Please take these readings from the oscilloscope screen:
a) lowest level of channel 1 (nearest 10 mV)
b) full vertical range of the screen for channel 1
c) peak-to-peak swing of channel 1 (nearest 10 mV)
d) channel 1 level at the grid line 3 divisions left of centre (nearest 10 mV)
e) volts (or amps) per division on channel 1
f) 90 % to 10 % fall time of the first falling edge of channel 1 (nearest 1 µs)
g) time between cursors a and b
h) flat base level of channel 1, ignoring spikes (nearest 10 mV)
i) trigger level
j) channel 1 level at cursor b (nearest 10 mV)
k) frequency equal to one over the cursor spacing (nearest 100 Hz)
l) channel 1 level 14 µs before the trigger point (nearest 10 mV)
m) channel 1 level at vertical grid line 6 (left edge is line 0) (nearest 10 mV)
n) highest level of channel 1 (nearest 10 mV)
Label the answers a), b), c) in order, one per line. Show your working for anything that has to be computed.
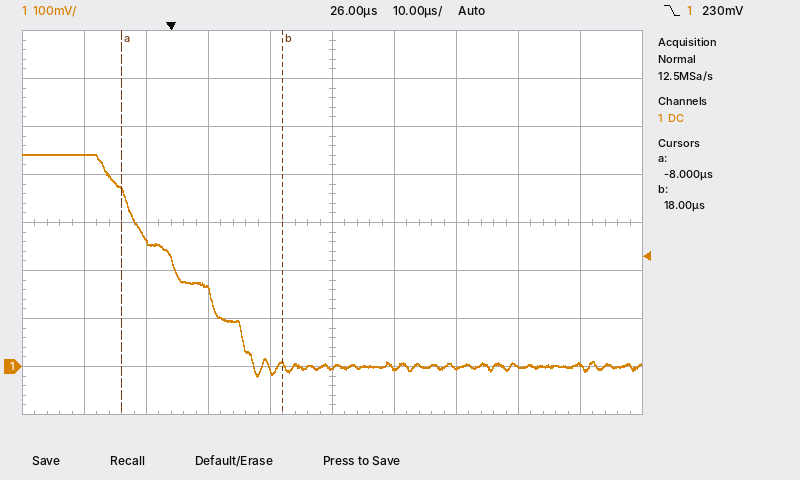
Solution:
a) -20 mV
b) 800 mV
c) 440 mV − (-20 mV) = 460 mV
d) 260 mV
e) 100 mV
f) 22 µs
g) 18 µs − (-8 µs) = 26 µs
h) 0 mV
i) 230 mV
j) 0 mV
k) 1 / 26 µs ≈ 38.5 kHz
l) 440 mV
m) 0 mV
n) 440 mV
